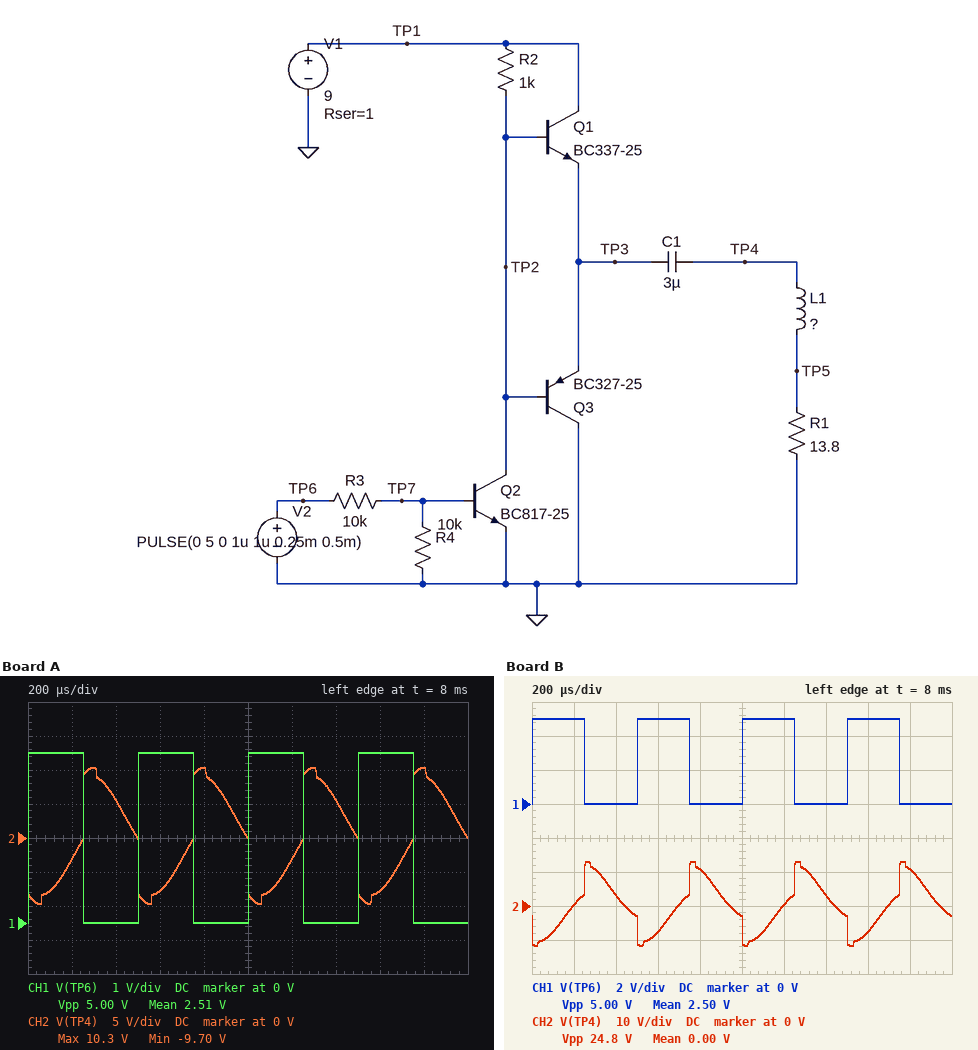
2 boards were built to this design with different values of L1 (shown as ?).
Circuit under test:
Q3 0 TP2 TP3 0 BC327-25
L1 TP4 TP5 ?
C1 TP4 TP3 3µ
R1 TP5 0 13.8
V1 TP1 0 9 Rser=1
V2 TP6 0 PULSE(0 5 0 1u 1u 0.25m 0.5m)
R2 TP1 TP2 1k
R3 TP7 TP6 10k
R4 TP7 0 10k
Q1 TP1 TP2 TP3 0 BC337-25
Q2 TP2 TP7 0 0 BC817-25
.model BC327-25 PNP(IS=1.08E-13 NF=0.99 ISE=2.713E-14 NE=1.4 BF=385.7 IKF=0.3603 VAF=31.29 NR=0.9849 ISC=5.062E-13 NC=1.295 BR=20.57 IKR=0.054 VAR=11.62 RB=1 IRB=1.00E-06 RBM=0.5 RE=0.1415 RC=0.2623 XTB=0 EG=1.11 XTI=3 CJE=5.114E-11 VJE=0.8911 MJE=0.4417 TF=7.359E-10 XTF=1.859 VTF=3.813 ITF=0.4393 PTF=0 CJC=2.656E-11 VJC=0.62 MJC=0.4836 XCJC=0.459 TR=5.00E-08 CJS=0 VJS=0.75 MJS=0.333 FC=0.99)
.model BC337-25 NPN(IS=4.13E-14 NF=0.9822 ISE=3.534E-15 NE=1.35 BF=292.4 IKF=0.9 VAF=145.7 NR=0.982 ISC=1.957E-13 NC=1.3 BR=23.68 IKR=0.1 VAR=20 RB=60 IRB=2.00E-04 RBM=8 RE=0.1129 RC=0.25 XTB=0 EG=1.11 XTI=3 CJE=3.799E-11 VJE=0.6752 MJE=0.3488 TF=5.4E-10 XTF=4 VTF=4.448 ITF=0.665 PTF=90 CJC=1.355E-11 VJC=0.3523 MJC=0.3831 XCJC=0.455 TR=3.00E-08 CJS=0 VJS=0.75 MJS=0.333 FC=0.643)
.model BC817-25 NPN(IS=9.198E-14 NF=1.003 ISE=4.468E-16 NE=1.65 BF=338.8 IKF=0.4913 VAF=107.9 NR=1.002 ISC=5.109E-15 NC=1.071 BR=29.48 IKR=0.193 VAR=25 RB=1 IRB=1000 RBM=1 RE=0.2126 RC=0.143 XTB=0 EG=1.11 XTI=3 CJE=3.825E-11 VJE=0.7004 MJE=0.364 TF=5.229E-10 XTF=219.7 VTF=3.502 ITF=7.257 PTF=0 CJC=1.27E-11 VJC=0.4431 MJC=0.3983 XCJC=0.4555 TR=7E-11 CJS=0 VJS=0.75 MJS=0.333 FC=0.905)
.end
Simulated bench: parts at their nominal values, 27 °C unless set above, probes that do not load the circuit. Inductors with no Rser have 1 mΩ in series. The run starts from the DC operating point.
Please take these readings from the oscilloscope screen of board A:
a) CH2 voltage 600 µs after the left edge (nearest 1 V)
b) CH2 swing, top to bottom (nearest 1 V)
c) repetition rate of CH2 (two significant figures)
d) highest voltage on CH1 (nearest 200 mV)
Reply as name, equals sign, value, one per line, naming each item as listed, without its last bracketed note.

CH2 voltage 600 µs after the left edge = -8 V
CH2 swing, top to bottom = 20 V
repetition rate of CH2 = 2.0 kHz
highest voltage on CH1 = 5.0 V
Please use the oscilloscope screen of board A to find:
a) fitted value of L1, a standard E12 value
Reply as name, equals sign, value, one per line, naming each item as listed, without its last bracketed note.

fitted value of L1, a standard E12 value = 3.9 mH
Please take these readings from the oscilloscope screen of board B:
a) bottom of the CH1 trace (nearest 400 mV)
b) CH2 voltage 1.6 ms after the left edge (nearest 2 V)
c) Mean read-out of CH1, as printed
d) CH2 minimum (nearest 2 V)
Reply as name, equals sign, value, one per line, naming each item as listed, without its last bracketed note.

bottom of the CH1 trace = 0 V
CH2 voltage 1.6 ms after the left edge = -8 V
Mean read-out of CH1, as printed = 2.50 V
CH2 minimum = -12 V
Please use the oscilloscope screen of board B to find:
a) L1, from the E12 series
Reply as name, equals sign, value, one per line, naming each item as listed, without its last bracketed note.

L1, from the E12 series = 2.7 mH
